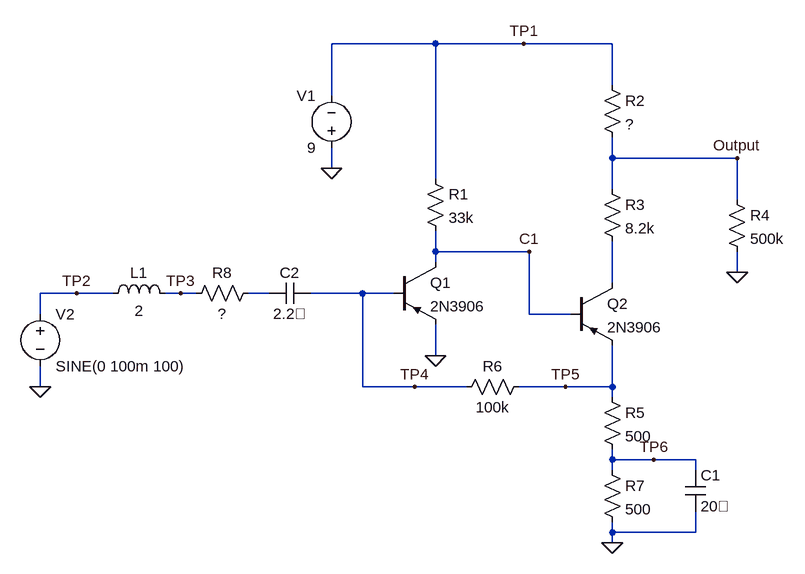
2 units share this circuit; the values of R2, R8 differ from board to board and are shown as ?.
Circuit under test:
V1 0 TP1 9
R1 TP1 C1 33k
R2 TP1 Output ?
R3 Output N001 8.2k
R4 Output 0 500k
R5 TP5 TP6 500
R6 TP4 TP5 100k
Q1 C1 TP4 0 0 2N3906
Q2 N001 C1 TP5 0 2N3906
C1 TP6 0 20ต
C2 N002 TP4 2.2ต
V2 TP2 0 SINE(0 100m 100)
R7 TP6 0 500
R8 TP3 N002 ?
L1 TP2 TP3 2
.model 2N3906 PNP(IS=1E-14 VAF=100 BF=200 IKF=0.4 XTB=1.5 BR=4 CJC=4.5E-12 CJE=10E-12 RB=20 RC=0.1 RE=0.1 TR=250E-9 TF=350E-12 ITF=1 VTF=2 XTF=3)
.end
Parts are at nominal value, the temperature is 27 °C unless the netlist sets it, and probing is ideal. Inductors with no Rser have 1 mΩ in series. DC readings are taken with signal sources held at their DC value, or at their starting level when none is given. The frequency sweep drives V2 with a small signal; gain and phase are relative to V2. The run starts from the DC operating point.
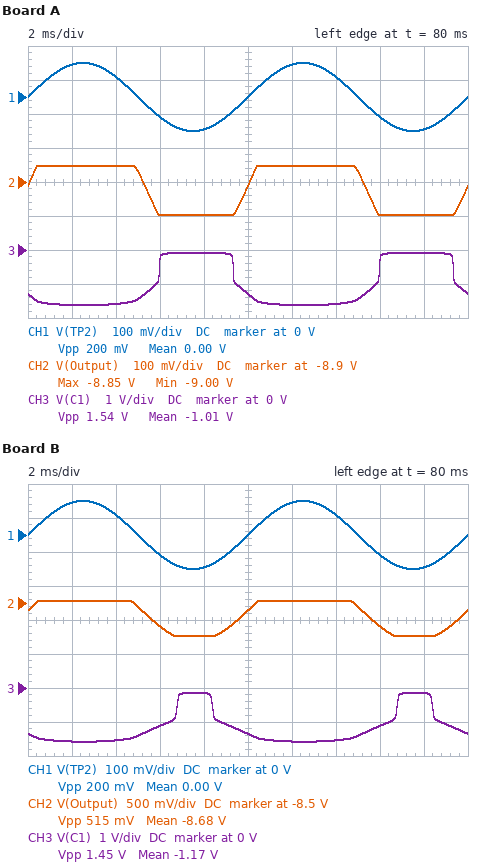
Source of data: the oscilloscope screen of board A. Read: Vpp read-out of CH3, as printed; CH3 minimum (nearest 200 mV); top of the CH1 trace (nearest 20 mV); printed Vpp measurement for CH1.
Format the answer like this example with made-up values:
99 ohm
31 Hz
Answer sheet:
1.54 V
-1.6 V
100 mV
200 mV
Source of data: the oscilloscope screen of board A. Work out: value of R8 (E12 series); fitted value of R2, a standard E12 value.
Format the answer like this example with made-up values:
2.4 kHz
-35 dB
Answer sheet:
12 kΩ
150 Ω
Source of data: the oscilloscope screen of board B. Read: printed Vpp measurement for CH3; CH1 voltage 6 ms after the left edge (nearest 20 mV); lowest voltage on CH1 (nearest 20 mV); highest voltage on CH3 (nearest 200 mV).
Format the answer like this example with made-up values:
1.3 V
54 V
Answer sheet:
1.45 V
-60 mV
-100 mV
-200 mV
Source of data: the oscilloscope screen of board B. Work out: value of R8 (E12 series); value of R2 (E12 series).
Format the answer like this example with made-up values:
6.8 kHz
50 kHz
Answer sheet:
22 kΩ
560 Ω
